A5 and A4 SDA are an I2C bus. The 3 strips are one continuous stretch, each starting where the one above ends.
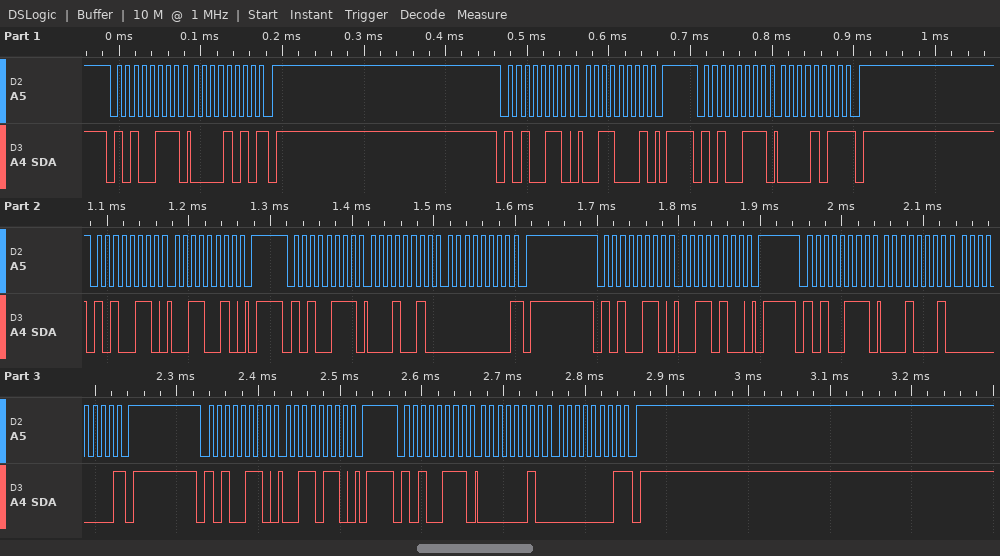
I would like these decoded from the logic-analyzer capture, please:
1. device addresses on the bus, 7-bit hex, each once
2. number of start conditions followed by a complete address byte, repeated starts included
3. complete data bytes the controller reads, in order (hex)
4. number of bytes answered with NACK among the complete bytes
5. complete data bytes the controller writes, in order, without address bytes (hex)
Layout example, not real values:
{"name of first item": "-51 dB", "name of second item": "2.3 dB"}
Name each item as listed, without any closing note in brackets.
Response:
{"device addresses on the bus, 7-bit hex, each once": "0x53", "number of start conditions followed by a complete address byte, repeated starts included": "9", "complete data bytes the controller reads, in order": "0A 0B 12 00 11 00 02 01", "number of bytes answered with NACK among the complete bytes": "5", "complete data bytes the controller writes, in order, without address bytes": "31 32 34 36"}
